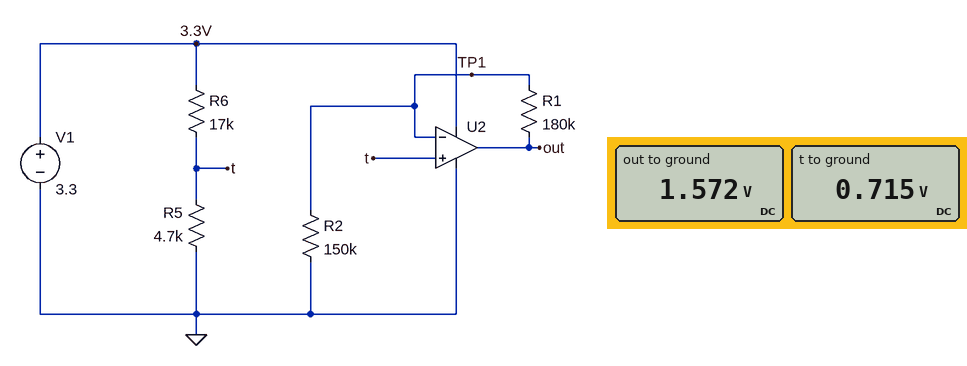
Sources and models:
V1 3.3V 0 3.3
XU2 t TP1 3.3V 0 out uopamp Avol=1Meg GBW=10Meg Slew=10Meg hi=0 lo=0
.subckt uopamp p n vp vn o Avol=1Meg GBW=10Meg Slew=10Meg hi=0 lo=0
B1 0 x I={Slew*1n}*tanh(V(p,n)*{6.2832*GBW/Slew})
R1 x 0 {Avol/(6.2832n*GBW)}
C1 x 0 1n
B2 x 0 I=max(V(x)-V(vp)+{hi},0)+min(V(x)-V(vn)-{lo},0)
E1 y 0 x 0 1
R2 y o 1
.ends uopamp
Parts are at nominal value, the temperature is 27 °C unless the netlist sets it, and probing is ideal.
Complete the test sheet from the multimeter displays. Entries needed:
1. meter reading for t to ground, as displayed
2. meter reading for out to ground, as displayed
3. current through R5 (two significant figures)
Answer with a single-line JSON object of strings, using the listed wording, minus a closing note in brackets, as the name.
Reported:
{"meter reading for t to ground, as displayed": "0.715 V", "meter reading for out to ground, as displayed": "1.572 V", "current through R5": "150 µA"}
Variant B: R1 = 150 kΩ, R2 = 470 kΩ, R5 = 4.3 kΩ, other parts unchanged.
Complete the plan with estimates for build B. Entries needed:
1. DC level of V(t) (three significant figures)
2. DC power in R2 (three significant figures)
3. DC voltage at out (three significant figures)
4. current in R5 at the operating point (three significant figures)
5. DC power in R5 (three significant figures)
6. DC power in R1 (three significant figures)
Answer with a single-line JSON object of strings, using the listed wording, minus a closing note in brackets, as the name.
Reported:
{"DC level of V(t)": "666 mV", "DC power in R2": "944 nW", "DC voltage at out": "879 mV", "current in R5 at the operating point": "155 µA", "DC power in R5": "103 µW", "DC power in R1": "301 nW"}
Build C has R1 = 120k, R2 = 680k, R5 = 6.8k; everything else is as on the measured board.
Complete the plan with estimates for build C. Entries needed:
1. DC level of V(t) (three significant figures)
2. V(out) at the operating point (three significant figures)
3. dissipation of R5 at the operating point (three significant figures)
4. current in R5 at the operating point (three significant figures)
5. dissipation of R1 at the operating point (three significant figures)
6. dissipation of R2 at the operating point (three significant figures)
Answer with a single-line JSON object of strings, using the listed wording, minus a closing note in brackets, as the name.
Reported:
{"DC level of V(t)": "943 mV", "V(out) at the operating point": "1.11 V", "dissipation of R5 at the operating point": "131 µW", "current in R5 at the operating point": "139 µA", "dissipation of R1 at the operating point": "231 nW", "dissipation of R2 at the operating point": "1.31 µW"}
